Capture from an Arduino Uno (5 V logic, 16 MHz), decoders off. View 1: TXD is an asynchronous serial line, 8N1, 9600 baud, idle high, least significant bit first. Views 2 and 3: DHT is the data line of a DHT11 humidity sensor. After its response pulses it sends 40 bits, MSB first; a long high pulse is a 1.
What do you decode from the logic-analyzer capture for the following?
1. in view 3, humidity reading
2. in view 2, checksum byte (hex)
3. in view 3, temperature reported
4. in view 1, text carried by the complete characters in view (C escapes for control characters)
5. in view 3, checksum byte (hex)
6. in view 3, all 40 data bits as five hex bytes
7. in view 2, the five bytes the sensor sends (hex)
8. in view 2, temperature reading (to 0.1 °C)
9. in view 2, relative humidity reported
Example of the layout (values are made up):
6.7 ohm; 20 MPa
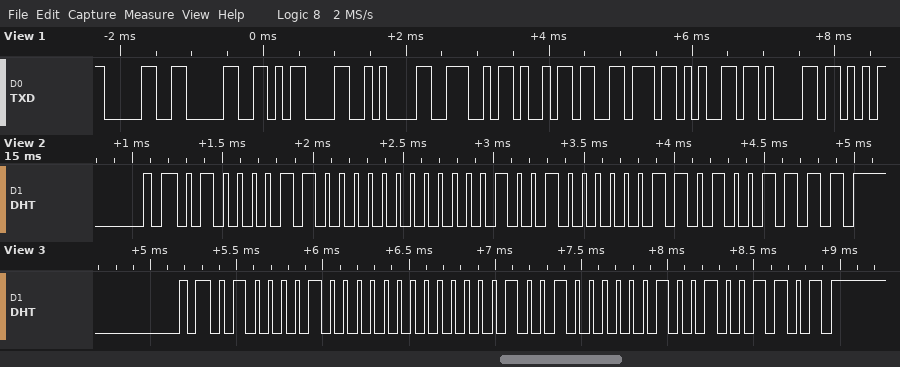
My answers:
66 %; 0x4F; 9.2 °C; "00\r\nNivea"; 0x4D; 42 00 09 02 4D; 43 00 09 03 4F; 9.3 °C; 67 %
